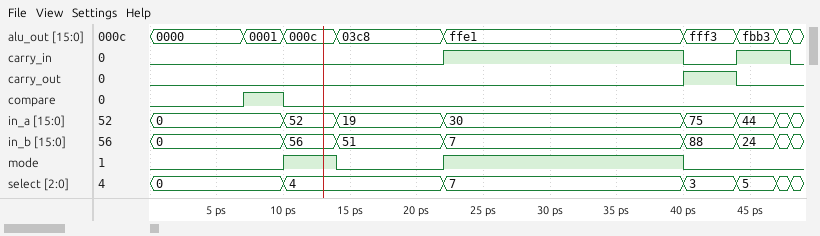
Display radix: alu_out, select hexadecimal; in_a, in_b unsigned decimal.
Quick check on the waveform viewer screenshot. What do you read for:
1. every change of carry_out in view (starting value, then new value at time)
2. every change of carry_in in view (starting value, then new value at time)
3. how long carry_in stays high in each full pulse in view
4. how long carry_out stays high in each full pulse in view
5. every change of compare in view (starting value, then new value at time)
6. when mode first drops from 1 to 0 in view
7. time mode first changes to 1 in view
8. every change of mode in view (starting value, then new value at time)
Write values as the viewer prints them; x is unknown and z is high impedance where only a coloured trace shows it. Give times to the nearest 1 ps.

0, 1 at 40 ps, 0 at 44 ps
0, 1 at 22 ps, 0 at 40 ps, 1 at 44 ps, 0 at 48 ps
18 ps, 4 ps
4 ps
0, 1 at 7 ps, 0 at 10 ps
14 ps
10 ps
0, 1 at 10 ps, 0 at 14 ps, 1 at 22 ps, 0 at 40 ps
